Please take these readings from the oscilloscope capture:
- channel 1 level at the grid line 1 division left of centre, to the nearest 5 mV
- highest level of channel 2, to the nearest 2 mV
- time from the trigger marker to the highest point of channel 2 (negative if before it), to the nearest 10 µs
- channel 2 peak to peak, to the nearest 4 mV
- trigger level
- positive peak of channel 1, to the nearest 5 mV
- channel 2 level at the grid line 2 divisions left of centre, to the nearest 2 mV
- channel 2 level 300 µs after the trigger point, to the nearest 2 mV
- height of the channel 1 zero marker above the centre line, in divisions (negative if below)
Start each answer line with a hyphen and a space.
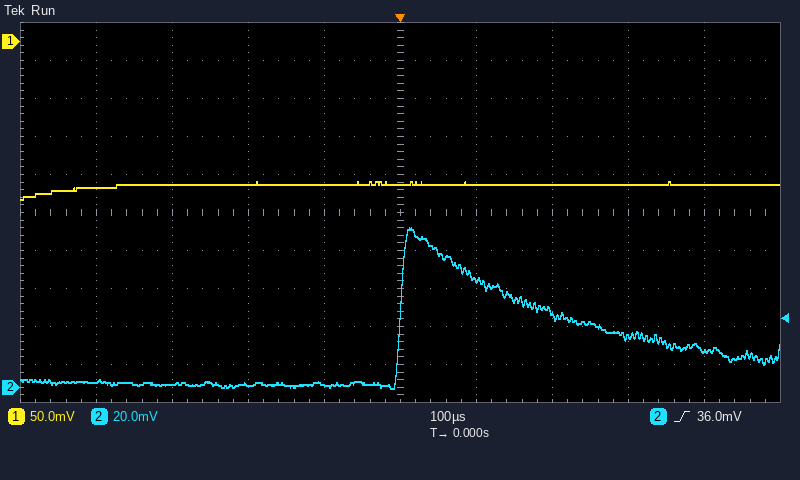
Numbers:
- -190 mV
- 84 mV
- +10 µs
- 84 mV
- 36.0 mV
- -185 mV
- 2 mV
- 26 mV
- +4.5 div
